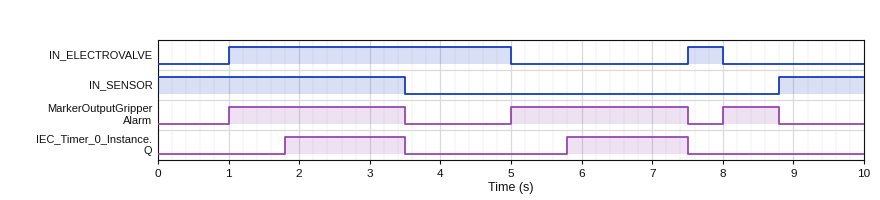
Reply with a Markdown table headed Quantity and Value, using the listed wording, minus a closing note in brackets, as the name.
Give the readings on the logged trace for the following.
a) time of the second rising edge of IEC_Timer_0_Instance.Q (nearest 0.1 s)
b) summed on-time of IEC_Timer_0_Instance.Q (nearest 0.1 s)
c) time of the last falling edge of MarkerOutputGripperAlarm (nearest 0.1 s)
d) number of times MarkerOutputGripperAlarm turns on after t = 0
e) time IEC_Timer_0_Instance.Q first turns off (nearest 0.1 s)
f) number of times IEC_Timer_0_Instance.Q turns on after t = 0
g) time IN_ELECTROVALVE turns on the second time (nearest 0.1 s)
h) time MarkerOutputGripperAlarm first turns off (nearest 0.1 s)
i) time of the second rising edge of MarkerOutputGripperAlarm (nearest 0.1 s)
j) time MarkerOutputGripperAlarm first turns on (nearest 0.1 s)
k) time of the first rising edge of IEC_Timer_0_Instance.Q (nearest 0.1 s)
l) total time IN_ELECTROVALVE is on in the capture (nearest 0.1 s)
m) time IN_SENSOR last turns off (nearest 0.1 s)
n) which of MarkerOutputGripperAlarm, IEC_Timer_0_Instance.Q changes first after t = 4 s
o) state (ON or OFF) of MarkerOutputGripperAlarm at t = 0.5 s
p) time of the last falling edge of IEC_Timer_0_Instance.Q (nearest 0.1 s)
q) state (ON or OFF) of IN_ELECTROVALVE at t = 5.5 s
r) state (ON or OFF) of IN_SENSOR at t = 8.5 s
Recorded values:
| Quantity | Value |
|---|---|
| time of the second rising edge of IEC_Timer_0_Instance.Q | 5.8 s |
| summed on-time of IEC_Timer_0_Instance.Q | 3.4 s |
| time of the last falling edge of MarkerOutputGripperAlarm | 8.8 s |
| number of times MarkerOutputGripperAlarm turns on after t = 0 | 3 |
| time IEC_Timer_0_Instance.Q first turns off | 3.5 s |
| number of times IEC_Timer_0_Instance.Q turns on after t = 0 | 2 |
| time IN_ELECTROVALVE turns on the second time | 7.5 s |
| time MarkerOutputGripperAlarm first turns off | 3.5 s |
| time of the second rising edge of MarkerOutputGripperAlarm | 5.0 s |
| time MarkerOutputGripperAlarm first turns on | 1.0 s |
| time of the first rising edge of IEC_Timer_0_Instance.Q | 1.8 s |
| total time IN_ELECTROVALVE is on in the capture | 4.5 s |
| time IN_SENSOR last turns off | 3.5 s |
| which of MarkerOutputGripperAlarm, IEC_Timer_0_Instance.Q changes first after t = 4 s | MarkerOutputGripperAlarm |
| state (ON or OFF) of MarkerOutputGripperAlarm at t = 0.5 s | OFF |
| time of the last falling edge of IEC_Timer_0_Instance.Q | 7.5 s |
| state (ON or OFF) of IN_ELECTROVALVE at t = 5.5 s | OFF |
| state (ON or OFF) of IN_SENSOR at t = 8.5 s | OFF |
